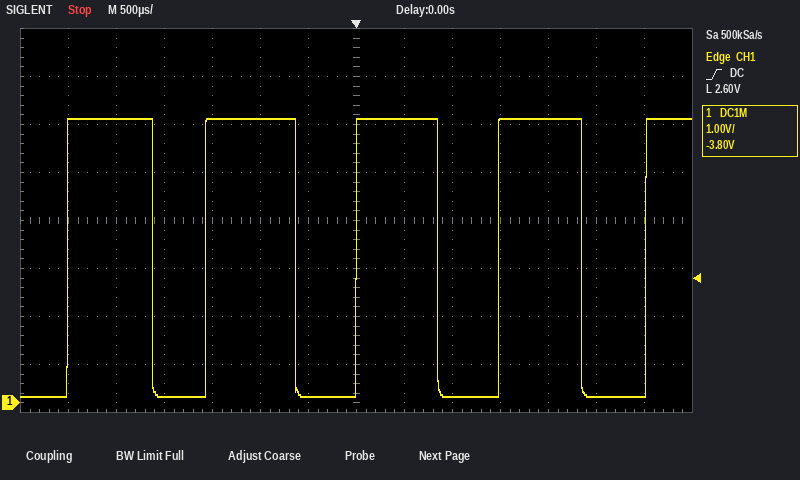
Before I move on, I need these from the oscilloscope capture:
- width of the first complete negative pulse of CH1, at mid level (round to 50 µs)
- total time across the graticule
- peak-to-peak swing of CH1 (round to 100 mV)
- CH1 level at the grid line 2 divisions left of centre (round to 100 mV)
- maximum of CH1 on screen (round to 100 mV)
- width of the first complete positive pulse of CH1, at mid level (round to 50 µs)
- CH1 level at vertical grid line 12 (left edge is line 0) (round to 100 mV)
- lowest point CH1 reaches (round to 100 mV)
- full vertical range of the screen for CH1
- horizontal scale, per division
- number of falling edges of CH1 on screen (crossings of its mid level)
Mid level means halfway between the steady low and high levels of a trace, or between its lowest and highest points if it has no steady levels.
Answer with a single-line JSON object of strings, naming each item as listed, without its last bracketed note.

{"width of the first complete negative pulse of CH1, at mid level": "550 µs", "total time across the graticule": "7 ms", "peak-to-peak swing of CH1": "5.8 V", "CH1 level at the grid line 2 divisions left of centre": "5.9 V", "maximum of CH1 on screen": "5.9 V", "width of the first complete positive pulse of CH1, at mid level": "900 µs", "CH1 level at vertical grid line 12 (left edge is line 0)": "100 mV", "lowest point CH1 reaches": "100 mV", "full vertical range of the screen for CH1": "8 V", "horizontal scale, per division": "500 µs", "number of falling edges of CH1 on screen": "4"}
